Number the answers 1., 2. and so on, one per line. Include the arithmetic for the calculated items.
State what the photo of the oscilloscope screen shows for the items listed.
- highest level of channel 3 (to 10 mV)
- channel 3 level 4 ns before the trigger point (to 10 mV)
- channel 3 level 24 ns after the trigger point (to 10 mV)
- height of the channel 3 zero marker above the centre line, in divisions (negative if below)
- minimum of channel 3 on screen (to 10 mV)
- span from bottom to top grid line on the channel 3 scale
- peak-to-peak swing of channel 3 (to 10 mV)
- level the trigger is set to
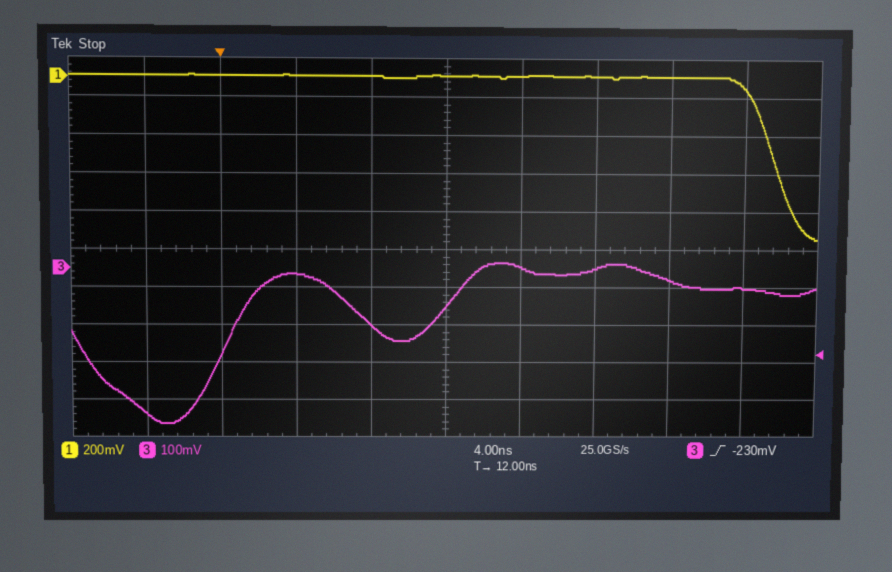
1. 20 mV
2. -390 mV
3. -30 mV
4. -0.5 div
5. -410 mV
6. 1 V
7. 20 mV − (-410 mV) = 430 mV
8. -230 mV
